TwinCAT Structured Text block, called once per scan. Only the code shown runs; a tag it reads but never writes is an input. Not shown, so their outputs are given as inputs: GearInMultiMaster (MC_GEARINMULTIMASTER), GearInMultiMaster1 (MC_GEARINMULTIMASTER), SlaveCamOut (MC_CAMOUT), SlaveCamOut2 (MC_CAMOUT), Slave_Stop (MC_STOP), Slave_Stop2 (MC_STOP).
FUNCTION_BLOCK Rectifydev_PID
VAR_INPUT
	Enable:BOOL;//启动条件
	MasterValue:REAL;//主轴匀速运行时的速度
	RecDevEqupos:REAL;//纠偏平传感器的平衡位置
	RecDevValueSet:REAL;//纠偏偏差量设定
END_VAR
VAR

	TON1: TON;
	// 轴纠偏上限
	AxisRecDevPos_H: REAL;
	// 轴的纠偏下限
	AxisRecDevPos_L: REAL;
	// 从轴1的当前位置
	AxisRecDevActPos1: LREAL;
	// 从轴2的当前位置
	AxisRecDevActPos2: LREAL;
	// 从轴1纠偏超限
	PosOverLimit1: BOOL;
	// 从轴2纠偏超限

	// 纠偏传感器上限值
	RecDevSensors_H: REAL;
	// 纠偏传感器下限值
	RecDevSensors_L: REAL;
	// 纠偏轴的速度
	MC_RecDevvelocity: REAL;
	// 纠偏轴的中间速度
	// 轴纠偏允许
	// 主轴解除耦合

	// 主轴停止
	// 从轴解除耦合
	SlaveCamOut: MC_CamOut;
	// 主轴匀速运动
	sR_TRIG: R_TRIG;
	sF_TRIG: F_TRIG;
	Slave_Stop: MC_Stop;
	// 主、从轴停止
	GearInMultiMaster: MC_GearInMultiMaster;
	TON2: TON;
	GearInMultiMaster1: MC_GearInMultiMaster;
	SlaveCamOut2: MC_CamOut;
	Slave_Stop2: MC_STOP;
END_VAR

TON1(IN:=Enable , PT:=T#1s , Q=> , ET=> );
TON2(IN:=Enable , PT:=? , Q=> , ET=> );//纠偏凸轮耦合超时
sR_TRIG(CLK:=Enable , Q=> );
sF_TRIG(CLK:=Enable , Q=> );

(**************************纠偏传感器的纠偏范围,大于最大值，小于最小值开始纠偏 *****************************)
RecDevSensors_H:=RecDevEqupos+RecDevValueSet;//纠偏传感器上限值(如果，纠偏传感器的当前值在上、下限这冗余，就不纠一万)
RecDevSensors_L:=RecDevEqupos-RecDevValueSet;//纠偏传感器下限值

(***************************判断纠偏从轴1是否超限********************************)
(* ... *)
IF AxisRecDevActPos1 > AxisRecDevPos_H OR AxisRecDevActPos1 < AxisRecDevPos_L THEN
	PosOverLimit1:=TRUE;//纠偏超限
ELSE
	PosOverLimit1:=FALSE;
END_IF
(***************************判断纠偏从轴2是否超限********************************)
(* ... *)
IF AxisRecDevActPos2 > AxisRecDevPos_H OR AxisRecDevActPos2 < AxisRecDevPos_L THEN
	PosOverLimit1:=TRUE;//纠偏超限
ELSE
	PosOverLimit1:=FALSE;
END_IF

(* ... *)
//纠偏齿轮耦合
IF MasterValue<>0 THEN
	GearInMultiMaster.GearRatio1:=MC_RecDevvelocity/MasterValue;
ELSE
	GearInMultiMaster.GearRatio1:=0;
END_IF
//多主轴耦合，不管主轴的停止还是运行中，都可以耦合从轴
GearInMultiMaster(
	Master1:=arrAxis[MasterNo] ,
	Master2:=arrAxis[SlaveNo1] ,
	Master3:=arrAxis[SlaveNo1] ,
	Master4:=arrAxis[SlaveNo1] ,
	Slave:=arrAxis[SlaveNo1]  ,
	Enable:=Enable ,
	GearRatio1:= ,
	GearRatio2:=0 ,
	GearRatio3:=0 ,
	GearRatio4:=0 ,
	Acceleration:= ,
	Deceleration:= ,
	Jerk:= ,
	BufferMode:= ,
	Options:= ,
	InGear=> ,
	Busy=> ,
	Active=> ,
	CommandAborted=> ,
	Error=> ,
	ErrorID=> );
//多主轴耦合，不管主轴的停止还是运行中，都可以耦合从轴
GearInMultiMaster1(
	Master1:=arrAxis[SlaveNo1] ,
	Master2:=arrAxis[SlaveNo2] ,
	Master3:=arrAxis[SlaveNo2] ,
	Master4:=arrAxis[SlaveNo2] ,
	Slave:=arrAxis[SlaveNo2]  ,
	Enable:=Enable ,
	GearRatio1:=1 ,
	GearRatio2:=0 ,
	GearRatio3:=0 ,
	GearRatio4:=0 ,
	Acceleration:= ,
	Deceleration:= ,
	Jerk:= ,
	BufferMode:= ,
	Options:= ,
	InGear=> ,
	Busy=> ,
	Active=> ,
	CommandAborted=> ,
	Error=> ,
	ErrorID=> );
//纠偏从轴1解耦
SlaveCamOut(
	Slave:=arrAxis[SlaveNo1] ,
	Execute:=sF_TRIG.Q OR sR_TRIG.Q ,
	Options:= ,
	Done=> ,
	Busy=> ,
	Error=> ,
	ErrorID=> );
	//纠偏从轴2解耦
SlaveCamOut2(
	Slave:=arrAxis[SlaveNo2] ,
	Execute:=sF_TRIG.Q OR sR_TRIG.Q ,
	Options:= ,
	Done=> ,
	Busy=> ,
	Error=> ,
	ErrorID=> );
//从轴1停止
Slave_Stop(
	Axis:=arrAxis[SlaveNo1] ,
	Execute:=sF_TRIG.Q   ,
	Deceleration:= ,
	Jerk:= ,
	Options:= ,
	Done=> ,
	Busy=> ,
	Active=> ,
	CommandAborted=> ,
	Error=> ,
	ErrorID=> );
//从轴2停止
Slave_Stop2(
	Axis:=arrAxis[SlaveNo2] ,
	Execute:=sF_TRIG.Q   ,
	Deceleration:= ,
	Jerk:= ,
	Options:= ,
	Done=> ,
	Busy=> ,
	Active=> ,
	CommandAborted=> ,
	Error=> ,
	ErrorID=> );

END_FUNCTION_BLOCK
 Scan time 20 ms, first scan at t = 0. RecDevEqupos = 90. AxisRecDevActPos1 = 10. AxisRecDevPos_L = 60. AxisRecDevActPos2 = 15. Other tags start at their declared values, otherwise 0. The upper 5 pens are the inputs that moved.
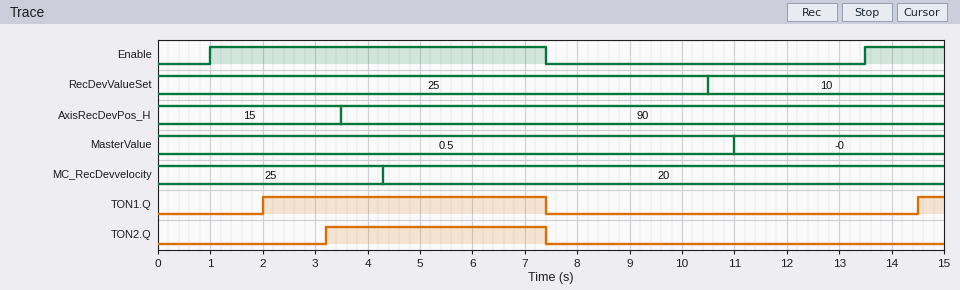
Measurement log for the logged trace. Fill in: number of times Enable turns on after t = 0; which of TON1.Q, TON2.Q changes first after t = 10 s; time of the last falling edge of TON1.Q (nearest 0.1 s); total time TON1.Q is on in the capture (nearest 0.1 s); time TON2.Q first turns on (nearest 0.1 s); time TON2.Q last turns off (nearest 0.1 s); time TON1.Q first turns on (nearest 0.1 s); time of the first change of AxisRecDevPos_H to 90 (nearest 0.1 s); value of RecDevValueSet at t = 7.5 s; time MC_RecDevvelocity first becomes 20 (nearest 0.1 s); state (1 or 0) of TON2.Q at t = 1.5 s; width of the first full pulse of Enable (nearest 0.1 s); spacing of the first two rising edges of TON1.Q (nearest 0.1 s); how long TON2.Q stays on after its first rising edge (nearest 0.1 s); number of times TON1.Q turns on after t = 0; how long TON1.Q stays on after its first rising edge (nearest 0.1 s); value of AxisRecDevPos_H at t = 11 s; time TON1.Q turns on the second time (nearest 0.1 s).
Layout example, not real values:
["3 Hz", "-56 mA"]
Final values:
["2", "TON1.Q", "7.4 s", "5.9 s", "3.2 s", "7.4 s", "2.0 s", "3.5 s", "25", "4.3 s", "0", "6.4 s", "12.5 s", "4.2 s", "2", "5.4 s", "90", "14.5 s"]
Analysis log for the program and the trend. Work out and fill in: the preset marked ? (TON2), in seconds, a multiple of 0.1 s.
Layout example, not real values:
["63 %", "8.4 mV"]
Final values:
["2.2 s"]
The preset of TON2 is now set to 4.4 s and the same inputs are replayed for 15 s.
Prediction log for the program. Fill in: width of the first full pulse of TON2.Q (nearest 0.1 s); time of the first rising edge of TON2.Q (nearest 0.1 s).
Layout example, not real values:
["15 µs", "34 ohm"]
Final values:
["2.0 s", "5.4 s"]
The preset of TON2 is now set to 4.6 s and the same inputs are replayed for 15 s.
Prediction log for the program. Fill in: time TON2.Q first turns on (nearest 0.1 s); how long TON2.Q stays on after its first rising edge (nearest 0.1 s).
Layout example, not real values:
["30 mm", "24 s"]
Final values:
["5.6 s", "1.8 s"]
